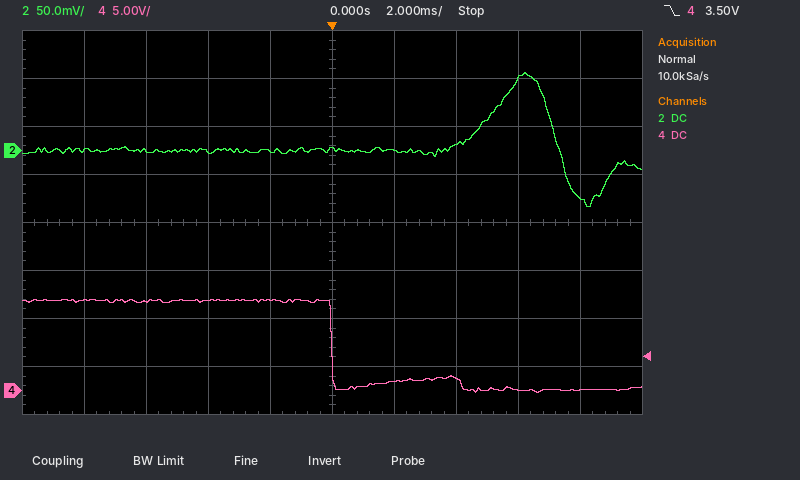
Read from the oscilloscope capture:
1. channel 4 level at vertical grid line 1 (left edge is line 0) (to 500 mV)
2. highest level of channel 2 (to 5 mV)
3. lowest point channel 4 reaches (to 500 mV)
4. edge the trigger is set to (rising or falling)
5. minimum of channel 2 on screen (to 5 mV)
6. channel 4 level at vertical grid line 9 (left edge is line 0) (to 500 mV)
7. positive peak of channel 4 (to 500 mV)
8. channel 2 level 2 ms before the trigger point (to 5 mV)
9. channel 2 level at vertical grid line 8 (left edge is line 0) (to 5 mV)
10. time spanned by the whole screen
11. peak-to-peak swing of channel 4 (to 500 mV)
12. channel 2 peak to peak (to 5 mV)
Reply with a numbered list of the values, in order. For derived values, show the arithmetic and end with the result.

1. 9.5 V
2. 80 mV
3. 0.0 V
4. falling
5. -60 mV
6. 0.0 V
7. 9.5 V
8. 0 mV
9. 75 mV
10. 20 ms
11. 9.5 V − (0.0 V) = 9.5 V
12. 80 mV − (-60 mV) = 140 mV
